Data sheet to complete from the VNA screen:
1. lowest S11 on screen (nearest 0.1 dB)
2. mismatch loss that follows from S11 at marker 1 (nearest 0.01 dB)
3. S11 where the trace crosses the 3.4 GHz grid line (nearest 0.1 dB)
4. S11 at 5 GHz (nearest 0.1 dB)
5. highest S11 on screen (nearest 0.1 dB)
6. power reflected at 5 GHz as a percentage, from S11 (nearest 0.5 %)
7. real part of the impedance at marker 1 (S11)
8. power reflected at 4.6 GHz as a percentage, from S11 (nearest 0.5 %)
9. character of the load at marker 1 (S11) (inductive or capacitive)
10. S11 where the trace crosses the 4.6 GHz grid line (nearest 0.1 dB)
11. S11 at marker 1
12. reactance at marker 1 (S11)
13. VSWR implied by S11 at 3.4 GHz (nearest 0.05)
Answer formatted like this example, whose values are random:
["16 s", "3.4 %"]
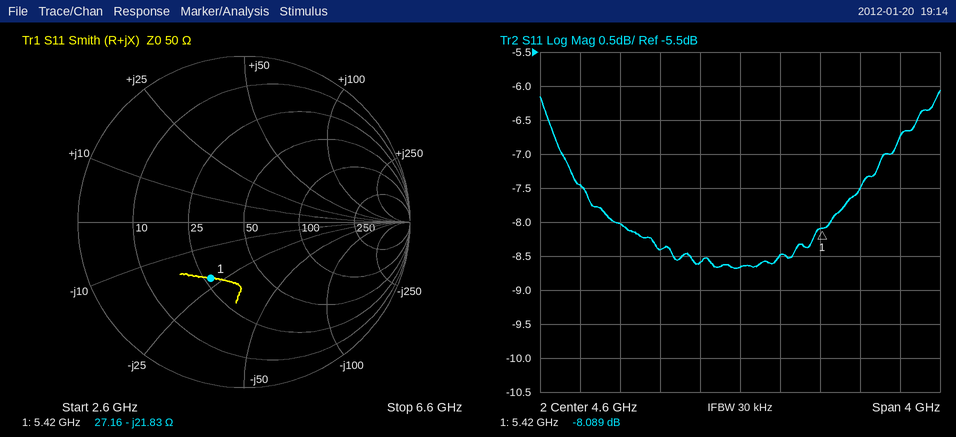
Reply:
["-8.7 dB", "0.73 dB", "-8.0 dB", "-8.5 dB", "-6.1 dB", "14.0 %", "27.16 Ω", "13.5 %", "capacitive", "-8.7 dB", "-8.089 dB", "-21.83 Ω", "2.30"]
